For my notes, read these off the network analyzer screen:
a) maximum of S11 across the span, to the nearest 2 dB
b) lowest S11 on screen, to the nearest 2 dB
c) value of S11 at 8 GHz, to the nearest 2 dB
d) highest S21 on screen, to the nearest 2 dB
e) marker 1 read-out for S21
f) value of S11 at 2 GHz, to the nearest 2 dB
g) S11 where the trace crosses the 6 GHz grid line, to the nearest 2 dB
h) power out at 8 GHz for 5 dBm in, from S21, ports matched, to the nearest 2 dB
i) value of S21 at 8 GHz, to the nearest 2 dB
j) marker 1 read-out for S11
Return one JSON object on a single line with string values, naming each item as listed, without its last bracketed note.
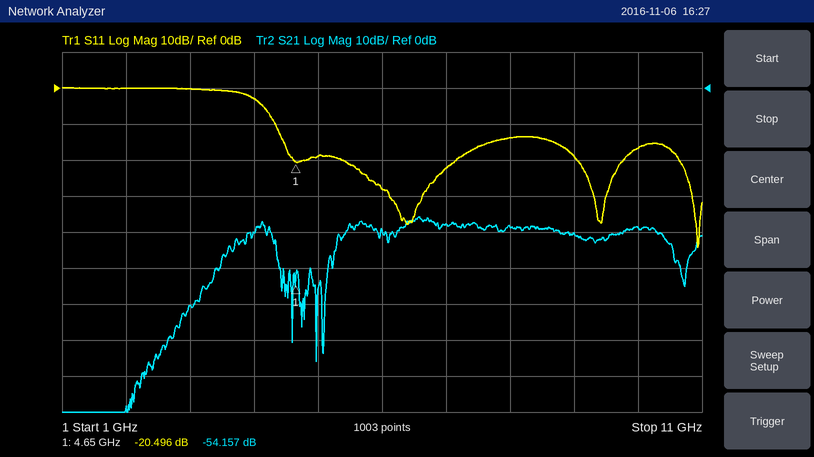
{"maximum of S11 across the span, to the nearest 2 dB": "0 dB", "lowest S11 on screen, to the nearest 2 dB": "-44 dB", "value of S11 at 8 GHz, to the nearest 2 dB": "-14 dB", "highest S21 on screen, to the nearest 2 dB": "-36 dB", "marker 1 read-out for S21": "-54.157 dB", "value of S11 at 2 GHz, to the nearest 2 dB": "0 dB", "S11 where the trace crosses the 6 GHz grid line, to the nearest 2 dB": "-28 dB", "power out at 8 GHz for 5 dBm in, from S21, ports matched, to the nearest 2 dB": "-34 dBm", "value of S21 at 8 GHz, to the nearest 2 dB": "-38 dB", "marker 1 read-out for S11": "-20.496 dB"}
